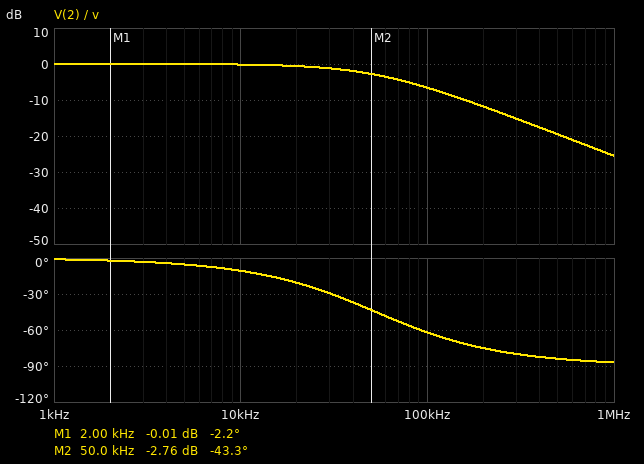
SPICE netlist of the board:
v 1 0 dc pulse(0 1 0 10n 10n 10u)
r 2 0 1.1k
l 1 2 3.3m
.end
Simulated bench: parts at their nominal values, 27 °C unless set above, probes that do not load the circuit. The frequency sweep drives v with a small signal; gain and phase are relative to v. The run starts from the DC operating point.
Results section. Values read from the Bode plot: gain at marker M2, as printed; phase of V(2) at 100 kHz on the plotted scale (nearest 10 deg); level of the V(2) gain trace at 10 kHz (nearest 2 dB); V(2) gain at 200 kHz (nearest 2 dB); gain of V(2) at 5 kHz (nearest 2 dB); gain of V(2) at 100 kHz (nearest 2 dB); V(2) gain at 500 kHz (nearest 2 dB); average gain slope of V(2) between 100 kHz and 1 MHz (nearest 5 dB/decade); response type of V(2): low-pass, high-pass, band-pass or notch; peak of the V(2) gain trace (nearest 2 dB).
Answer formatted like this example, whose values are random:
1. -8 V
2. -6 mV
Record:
1. -2.76 dB
2. -60 deg
3. 0 dB
4. -12 dB
5. 0 dB
6. -6 dB
7. -20 dB
8. -20 dB/decade
9. low-pass
10. 0 dB
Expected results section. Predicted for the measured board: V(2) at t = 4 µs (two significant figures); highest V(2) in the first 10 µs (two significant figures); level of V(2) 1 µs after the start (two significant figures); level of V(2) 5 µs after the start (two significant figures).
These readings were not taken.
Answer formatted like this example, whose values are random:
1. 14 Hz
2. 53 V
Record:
1. 740 mV
2. 960 mV
3. 280 mV
4. 810 mV
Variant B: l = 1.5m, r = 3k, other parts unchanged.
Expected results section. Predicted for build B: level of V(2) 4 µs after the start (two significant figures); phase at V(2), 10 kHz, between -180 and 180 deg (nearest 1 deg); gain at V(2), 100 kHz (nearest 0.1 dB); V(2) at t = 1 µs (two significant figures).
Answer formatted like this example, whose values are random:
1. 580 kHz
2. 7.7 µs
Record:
1. 1.0 V
2. -2 deg
3. -0.4 dB
4. 860 mV
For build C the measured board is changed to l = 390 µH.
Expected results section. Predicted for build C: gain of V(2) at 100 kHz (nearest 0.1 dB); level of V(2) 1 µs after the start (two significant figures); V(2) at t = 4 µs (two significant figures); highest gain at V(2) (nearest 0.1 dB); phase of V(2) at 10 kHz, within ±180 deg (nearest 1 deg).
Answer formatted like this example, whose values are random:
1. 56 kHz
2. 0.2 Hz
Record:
1. -0.2 dB
2. 940 mV
3. 1.0 V
4. 0 dB
5. -1 deg
